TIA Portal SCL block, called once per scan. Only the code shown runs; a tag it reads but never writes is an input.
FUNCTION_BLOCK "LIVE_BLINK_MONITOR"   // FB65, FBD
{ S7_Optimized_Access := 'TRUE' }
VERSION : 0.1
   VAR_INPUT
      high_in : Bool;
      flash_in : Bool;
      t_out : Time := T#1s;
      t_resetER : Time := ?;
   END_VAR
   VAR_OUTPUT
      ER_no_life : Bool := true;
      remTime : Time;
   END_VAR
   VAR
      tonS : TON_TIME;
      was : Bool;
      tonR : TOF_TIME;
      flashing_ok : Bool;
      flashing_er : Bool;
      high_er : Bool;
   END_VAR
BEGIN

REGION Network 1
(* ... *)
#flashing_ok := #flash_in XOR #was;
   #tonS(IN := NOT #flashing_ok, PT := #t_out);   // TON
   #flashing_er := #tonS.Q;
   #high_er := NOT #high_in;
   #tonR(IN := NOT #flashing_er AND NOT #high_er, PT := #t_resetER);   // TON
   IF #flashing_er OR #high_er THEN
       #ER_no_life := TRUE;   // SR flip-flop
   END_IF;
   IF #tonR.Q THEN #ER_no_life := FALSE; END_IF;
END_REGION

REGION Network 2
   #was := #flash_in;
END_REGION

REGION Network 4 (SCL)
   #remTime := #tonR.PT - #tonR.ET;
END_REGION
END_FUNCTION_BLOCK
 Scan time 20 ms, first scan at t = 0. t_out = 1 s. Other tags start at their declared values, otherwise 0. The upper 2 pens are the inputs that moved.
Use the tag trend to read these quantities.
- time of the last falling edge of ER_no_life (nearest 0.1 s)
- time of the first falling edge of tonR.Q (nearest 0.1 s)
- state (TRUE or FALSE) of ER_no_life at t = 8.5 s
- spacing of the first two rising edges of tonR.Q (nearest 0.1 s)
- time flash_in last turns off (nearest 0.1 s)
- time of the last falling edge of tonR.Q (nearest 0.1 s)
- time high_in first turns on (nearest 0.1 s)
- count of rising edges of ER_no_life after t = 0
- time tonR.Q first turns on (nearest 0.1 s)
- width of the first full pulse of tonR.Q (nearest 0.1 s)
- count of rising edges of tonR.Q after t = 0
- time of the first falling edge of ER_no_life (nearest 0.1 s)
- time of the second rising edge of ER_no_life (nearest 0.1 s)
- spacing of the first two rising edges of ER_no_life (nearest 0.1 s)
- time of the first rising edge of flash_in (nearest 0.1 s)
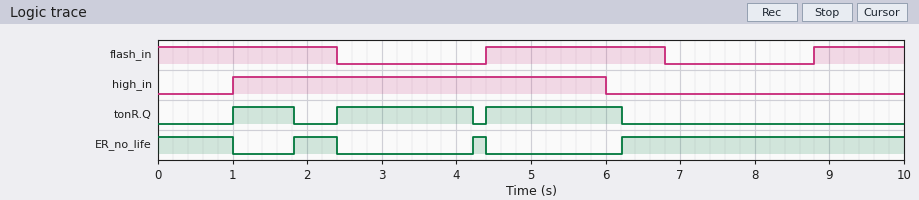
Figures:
4.4 s
1.8 s
TRUE
1.4 s
6.8 s
6.2 s
1.0 s
3
1.0 s
0.8 s
3
1.0 s
4.2 s
2.4 s
4.4 s
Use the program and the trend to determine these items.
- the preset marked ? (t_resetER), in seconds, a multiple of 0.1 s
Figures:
0.8 s
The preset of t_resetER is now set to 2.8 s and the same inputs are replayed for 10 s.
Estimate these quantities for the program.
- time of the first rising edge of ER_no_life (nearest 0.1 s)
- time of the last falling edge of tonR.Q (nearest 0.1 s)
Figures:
8.2 s
8.2 s
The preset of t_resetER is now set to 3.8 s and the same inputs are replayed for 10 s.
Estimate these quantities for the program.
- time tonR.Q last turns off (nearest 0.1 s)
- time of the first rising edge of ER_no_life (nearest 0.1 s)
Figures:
9.2 s
9.2 s
